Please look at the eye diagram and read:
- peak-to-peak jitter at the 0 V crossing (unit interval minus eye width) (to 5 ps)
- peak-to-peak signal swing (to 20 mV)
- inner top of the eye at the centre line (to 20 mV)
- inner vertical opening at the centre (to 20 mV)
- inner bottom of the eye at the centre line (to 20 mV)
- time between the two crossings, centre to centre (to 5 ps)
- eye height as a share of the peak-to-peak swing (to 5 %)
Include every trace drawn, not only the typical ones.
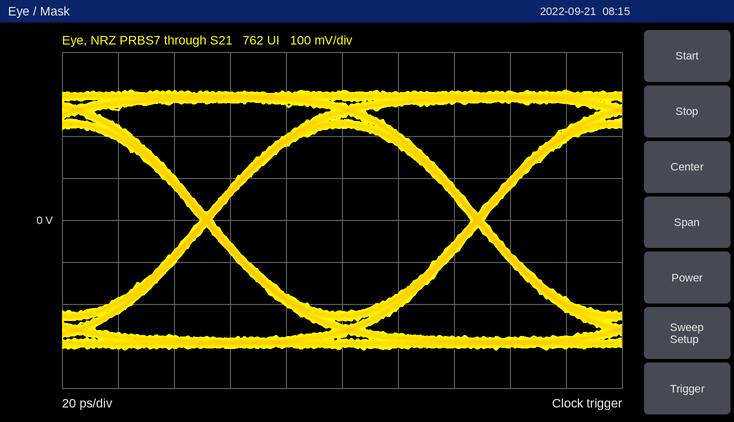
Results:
5 ps
620 mV
220 mV
440 mV
-220 mV
95 ps
70 %
